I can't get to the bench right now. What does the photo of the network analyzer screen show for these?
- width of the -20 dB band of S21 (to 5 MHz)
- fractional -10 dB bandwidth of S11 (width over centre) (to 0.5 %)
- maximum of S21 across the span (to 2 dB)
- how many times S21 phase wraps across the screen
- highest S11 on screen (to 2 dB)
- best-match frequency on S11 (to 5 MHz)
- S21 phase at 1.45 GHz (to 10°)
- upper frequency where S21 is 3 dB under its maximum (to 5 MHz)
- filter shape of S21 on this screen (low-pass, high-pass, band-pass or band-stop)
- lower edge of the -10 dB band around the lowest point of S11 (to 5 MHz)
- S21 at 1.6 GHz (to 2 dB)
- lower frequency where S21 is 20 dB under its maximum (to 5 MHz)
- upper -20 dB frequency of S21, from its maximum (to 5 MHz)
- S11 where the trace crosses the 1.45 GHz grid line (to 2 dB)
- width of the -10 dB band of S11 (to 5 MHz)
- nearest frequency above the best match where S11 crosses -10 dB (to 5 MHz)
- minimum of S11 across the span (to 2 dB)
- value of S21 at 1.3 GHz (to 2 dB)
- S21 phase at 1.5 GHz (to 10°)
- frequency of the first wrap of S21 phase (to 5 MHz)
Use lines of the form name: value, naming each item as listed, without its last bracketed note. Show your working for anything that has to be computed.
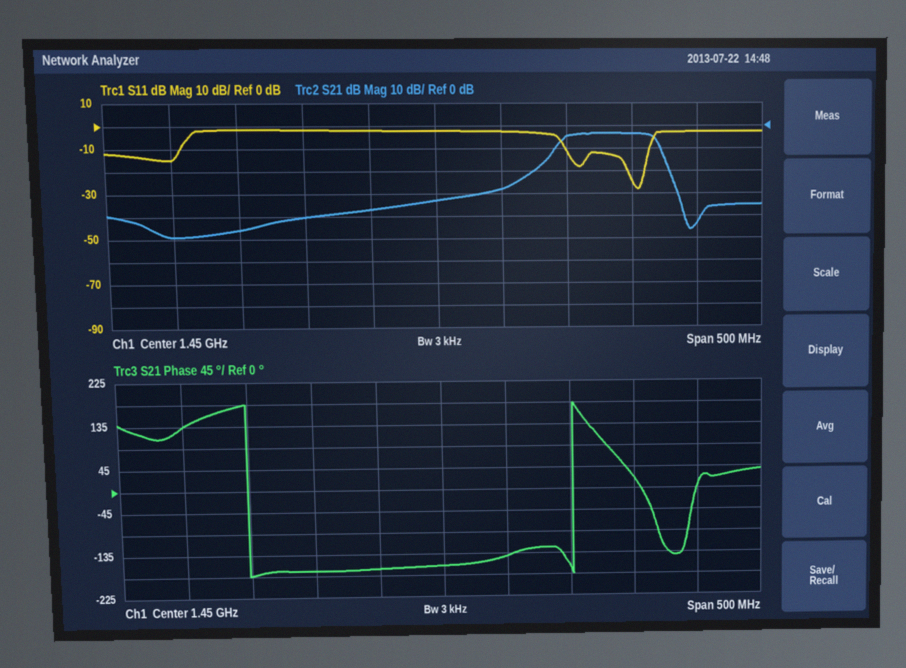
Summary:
width of the -20 dB band of S21: 1.630 GHz − 1.515 GHz = 115 MHz
fractional -10 dB bandwidth of S11 (width over centre): 65 MHz / 1.5825 GHz ≈ 4.11 %, so 4.0 % to the nearest 0.5 %
maximum of S21 across the span: -4 dB
how many times S21 phase wraps across the screen: 2
highest S11 on screen: -2 dB
best-match frequency on S11: 1.605 GHz
S21 phase at 1.45 GHz: -160°
upper frequency where S21 is 3 dB under its maximum: 1.620 GHz
filter shape of S21 on this screen: band-pass
lower edge of the -10 dB band around the lowest point of S11: 1.550 GHz
S21 at 1.6 GHz: -4 dB
lower frequency where S21 is 20 dB under its maximum: 1.515 GHz
upper -20 dB frequency of S21, from its maximum: 1.630 GHz
S11 where the trace crosses the 1.45 GHz grid line: -2 dB
width of the -10 dB band of S11: 1.615 GHz − 1.550 GHz = 65 MHz
nearest frequency above the best match where S11 crosses -10 dB: 1.615 GHz
minimum of S11 across the span: -28 dB
value of S21 at 1.3 GHz: -46 dB
S21 phase at 1.5 GHz: -140°
frequency of the first wrap of S21 phase: 1.300 GHz
